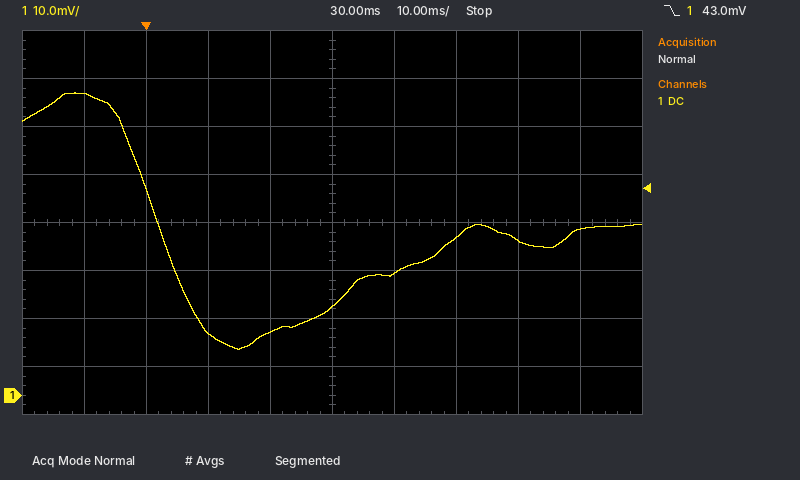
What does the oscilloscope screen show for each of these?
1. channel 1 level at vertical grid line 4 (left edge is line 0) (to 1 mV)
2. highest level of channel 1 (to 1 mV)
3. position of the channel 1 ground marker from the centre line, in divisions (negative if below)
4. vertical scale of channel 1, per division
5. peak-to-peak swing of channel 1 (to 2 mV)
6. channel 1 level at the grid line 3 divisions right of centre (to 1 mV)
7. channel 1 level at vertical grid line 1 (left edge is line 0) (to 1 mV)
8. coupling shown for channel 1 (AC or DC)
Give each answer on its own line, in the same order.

13 mV
63 mV
-3.6 div
10 mV
54 mV
32 mV
63 mV
DC
